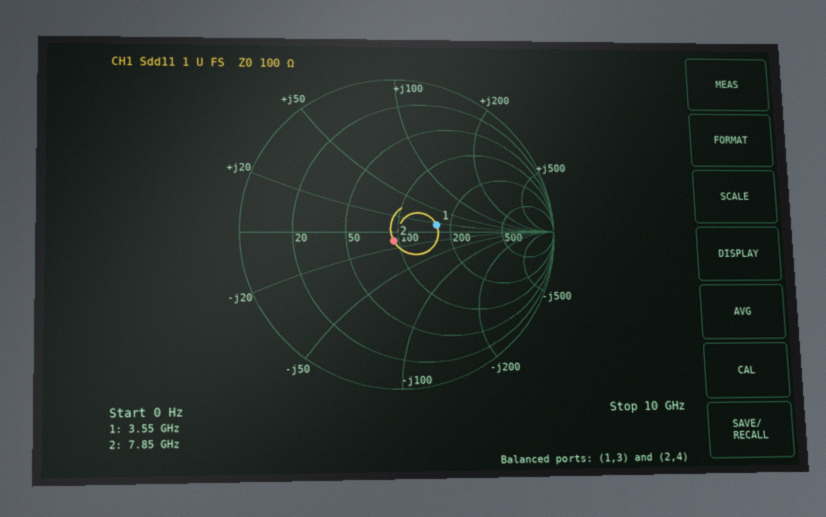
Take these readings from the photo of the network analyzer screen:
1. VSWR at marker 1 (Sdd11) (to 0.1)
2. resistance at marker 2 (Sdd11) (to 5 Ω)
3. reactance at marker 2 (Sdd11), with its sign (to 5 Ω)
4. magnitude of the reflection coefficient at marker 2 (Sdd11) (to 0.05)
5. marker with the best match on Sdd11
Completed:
1.7
95 Ω
-10 Ω
0.05
marker 2
